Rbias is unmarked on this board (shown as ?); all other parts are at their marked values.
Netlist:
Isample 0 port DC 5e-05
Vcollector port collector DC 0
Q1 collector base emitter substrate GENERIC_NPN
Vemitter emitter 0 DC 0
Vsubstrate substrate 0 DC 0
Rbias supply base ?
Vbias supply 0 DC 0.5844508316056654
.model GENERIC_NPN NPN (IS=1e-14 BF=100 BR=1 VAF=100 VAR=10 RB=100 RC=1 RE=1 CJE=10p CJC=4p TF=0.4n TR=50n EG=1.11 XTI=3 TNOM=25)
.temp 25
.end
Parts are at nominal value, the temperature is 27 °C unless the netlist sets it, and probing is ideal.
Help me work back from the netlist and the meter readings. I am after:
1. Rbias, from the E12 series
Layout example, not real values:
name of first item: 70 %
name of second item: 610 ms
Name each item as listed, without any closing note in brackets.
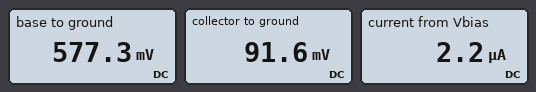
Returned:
Rbias, from the E12 series: 3.3 kΩ
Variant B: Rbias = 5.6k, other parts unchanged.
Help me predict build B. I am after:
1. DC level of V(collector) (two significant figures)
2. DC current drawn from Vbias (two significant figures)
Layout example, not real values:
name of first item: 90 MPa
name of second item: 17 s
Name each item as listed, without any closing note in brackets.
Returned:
DC level of V(collector): 110 mV
DC current drawn from Vbias: 1.4 µA
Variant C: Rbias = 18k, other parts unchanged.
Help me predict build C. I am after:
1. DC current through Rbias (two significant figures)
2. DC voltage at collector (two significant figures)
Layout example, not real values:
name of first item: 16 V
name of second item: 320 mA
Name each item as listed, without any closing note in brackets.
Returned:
DC current through Rbias: 520 nA
DC voltage at collector: 1.9 V
